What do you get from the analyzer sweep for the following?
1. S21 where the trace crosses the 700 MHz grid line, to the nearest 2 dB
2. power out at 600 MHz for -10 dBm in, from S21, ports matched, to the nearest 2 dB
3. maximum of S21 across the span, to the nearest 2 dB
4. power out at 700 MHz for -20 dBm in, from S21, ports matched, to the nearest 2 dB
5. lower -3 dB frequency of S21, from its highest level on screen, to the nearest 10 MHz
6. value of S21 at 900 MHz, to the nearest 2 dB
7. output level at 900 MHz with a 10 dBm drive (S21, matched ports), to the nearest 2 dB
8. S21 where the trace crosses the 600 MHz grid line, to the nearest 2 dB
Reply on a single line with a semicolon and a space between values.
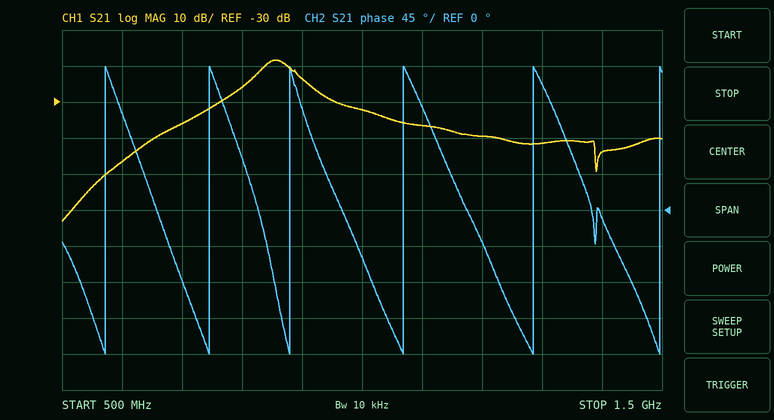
-36 dB; -56 dBm; -18 dB; -56 dBm; 830 MHz; -24 dB; -14 dBm; -46 dB
